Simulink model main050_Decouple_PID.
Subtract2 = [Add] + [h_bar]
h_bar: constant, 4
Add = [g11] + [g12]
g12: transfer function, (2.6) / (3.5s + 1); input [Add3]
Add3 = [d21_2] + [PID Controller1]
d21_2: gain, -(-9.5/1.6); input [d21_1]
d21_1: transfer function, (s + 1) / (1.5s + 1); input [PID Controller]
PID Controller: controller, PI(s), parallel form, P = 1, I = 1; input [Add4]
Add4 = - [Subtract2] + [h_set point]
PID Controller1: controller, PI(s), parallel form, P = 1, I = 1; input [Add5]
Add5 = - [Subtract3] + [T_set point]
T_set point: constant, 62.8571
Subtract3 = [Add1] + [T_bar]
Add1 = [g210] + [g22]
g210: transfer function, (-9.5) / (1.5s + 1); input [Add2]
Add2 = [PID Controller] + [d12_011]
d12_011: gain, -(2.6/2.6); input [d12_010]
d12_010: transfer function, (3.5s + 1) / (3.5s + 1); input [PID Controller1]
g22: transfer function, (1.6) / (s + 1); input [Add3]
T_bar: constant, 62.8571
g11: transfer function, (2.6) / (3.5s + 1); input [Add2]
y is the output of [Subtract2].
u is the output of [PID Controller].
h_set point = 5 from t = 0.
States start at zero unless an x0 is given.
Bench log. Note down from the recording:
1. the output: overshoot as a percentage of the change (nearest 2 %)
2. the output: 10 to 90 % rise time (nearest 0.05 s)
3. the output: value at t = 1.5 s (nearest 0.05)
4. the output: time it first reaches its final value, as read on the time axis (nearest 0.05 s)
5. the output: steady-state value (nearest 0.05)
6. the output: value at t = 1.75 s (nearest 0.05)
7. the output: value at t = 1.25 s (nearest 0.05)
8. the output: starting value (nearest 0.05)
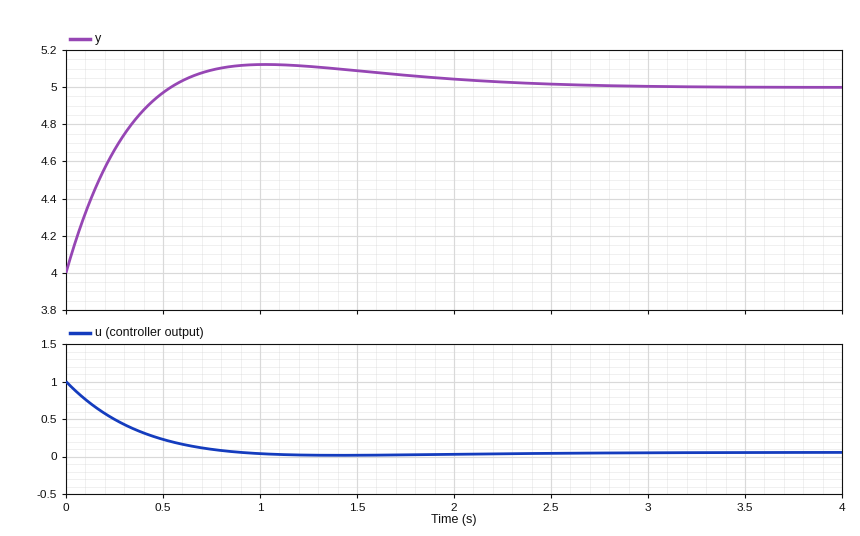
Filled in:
12 %
0.40 s
5.10
0.55 s
5.00
5.05
5.10
4.00
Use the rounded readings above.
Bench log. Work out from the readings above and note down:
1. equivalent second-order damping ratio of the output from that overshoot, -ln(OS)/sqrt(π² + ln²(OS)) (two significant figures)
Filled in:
0.56
